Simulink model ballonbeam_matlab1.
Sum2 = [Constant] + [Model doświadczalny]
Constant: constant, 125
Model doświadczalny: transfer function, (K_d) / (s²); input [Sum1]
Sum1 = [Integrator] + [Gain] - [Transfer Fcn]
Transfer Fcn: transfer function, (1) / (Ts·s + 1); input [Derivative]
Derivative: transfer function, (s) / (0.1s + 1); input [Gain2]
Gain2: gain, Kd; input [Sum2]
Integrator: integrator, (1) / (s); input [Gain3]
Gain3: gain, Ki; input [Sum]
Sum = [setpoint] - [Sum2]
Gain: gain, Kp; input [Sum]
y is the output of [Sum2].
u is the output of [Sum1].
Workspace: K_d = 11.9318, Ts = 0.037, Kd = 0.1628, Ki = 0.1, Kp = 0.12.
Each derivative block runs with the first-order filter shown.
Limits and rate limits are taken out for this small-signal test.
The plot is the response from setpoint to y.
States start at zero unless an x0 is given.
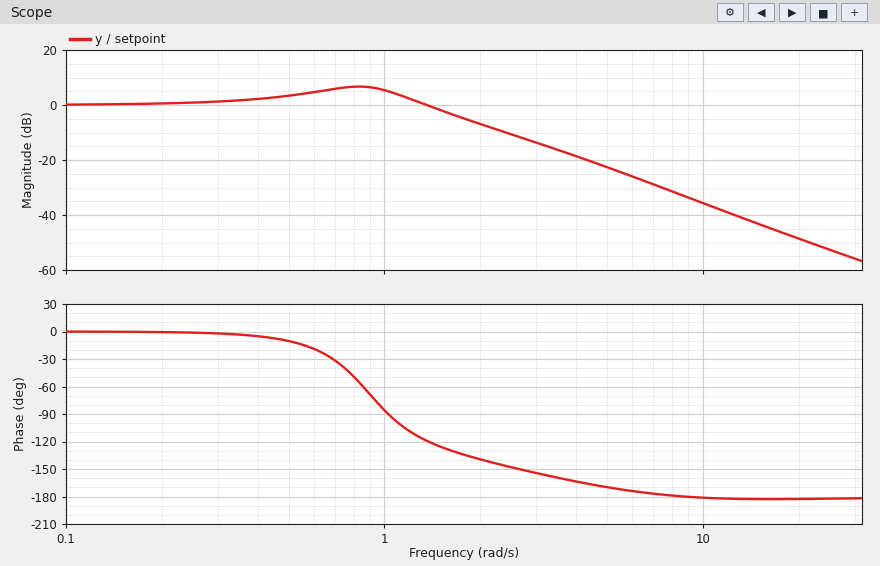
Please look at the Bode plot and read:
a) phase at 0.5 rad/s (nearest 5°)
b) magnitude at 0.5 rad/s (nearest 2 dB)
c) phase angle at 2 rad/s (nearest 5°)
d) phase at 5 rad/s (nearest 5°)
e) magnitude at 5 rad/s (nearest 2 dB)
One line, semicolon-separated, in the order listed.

-10°; 4 dB; -140°; -170°; -22 dB
